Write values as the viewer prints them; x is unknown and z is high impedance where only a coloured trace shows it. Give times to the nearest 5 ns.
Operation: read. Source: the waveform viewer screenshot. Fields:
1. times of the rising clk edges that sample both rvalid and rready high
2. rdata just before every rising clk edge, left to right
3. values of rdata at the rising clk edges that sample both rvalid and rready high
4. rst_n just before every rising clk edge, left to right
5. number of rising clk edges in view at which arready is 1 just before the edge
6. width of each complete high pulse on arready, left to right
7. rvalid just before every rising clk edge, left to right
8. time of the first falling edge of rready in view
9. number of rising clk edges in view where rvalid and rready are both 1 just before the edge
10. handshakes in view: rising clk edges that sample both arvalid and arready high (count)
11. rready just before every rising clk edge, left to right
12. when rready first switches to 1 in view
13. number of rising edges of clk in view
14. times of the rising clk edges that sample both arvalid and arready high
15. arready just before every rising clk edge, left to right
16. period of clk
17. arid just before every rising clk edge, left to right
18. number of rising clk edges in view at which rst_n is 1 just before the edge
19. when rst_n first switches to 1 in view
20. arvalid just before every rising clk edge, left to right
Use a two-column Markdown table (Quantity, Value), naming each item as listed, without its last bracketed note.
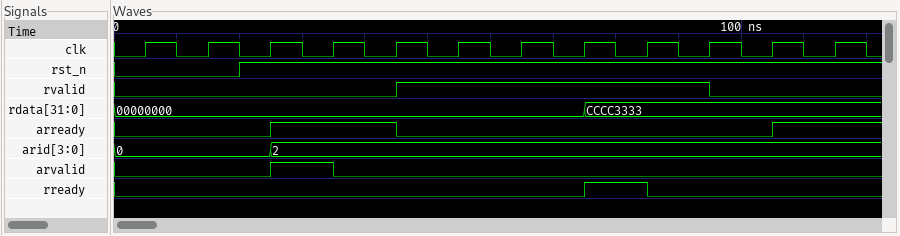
| Quantity | Value |
|---|---|
| times of the rising clk edges that sample both rvalid and rready high | 85 ns |
| rdata just before every rising clk edge, left to right | 00000000, 00000000, 00000000, 00000000, 00000000, 00000000, 00000000, 00000000, CCCC3333, CCCC3333, CCCC3333, CCCC3333 |
| values of rdata at the rising clk edges that sample both rvalid and rready high | CCCC3333 |
| rst_n just before every rising clk edge, left to right | 0 0 1 1 1 1 1 1 1 1 1 1 |
| number of rising clk edges in view at which arready is 1 just before the edge | 3 |
| width of each complete high pulse on arready, left to right | 20 ns |
| rvalid just before every rising clk edge, left to right | 0 0 0 0 0 1 1 1 1 1 0 0 |
| time of the first falling edge of rready in view | 85 ns |
| number of rising clk edges in view where rvalid and rready are both 1 just before the edge | 1 |
| handshakes in view: rising clk edges that sample both arvalid and arready high | 1 |
| rready just before every rising clk edge, left to right | 0 0 0 0 0 0 0 0 1 0 0 0 |
| when rready first switches to 1 in view | 75 ns |
| number of rising edges of clk in view | 12 |
| times of the rising clk edges that sample both arvalid and arready high | 35 ns |
| arready just before every rising clk edge, left to right | 0 0 0 1 1 0 0 0 0 0 0 1 |
| period of clk | 10 ns |
| arid just before every rising clk edge, left to right | 0, 0, 0, 2, 2, 2, 2, 2, 2, 2, 2, 2 |
| number of rising clk edges in view at which rst_n is 1 just before the edge | 10 |
| when rst_n first switches to 1 in view | 20 ns |
| arvalid just before every rising clk edge, left to right | 0 0 0 1 0 0 0 0 0 0 0 0 |
